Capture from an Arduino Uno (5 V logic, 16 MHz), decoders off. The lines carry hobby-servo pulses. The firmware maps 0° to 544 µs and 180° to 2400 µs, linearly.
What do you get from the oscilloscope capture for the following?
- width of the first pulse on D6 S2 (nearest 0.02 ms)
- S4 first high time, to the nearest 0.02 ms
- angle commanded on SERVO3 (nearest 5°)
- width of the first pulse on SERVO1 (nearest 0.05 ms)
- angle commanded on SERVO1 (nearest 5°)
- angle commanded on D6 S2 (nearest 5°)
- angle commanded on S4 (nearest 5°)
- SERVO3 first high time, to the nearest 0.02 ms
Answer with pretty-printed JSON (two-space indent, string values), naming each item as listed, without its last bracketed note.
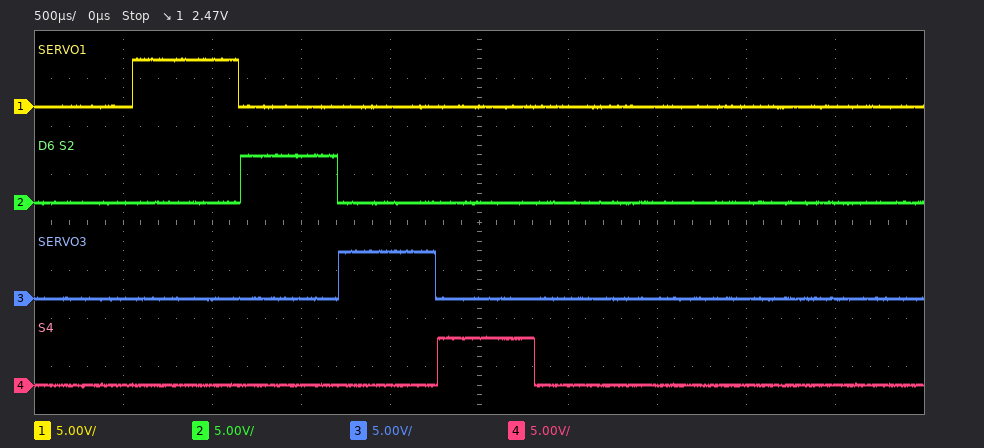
{
  "width of the first pulse on D6 S2": "0.54 ms",
  "S4 first high time, to the nearest 0.02 ms": "0.54 ms",
  "angle commanded on SERVO3": "0°",
  "width of the first pulse on SERVO1": "0.60 ms",
  "angle commanded on SERVO1": "5°",
  "angle commanded on D6 S2": "0°",
  "angle commanded on S4": "0°",
  "SERVO3 first high time, to the nearest 0.02 ms": "0.54 ms"
}
